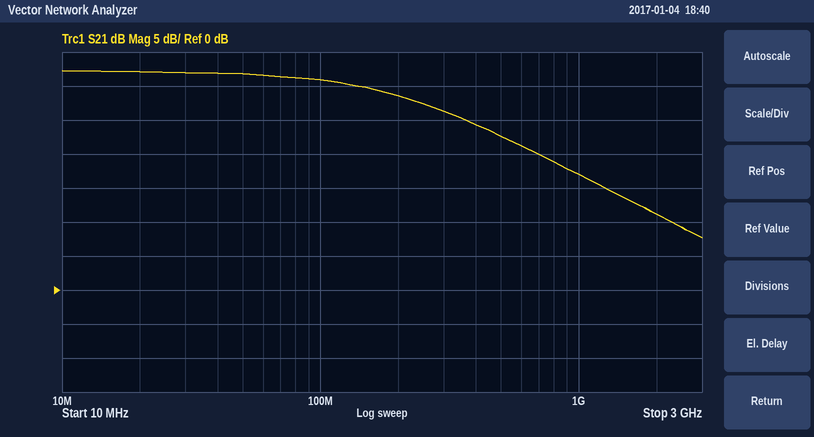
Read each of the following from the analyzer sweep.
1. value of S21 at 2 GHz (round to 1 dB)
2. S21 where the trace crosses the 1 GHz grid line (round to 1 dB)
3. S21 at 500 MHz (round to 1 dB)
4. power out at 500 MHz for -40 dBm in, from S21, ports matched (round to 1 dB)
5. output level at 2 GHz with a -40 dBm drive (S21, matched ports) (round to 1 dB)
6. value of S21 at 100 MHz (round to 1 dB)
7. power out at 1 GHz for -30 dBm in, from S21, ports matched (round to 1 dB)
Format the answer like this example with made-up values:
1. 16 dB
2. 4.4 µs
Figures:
1. 11 dB
2. 17 dB
3. 23 dB
4. -17 dBm
5. -29 dBm
6. 31 dB
7. -13 dBm
